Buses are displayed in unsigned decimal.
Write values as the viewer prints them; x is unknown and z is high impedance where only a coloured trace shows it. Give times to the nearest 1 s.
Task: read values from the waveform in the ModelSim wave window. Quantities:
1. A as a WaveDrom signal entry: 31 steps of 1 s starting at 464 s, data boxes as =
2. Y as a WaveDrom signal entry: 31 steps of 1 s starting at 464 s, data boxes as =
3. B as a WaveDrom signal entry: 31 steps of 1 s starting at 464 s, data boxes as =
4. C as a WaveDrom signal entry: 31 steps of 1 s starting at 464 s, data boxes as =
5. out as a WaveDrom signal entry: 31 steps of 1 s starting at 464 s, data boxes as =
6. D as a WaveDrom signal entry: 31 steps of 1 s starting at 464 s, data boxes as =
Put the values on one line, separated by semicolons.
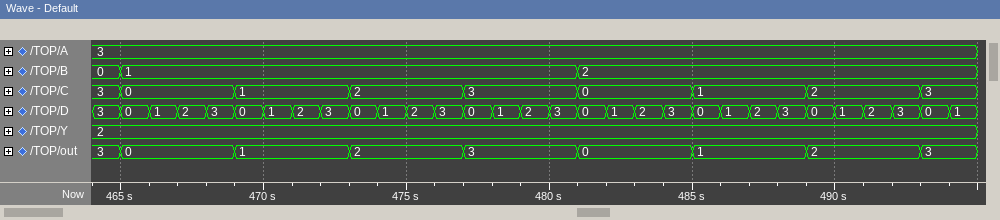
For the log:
{name: 'A', wave: '=..............................', data: '3'}; {name: 'Y', wave: '=..............................', data: '2'}; {name: 'B', wave: '==...............=.............', data: '0 1 2'}; {name: 'C', wave: '==...=...=...=...=...=...=...=.', data: '3 0 1 2 3 0 1 2 3'}; {name: 'out', wave: '==...=...=...=...=...=...=...=.', data: '3 0 1 2 3 0 1 2 3'}; {name: 'D', wave: '===============================', data: '3 0 1 2 3 0 1 2 3 0 1 2 3 0 1 2 3 0 1 2 3 0 1 2 3 0 1 2 3 0 1'}
